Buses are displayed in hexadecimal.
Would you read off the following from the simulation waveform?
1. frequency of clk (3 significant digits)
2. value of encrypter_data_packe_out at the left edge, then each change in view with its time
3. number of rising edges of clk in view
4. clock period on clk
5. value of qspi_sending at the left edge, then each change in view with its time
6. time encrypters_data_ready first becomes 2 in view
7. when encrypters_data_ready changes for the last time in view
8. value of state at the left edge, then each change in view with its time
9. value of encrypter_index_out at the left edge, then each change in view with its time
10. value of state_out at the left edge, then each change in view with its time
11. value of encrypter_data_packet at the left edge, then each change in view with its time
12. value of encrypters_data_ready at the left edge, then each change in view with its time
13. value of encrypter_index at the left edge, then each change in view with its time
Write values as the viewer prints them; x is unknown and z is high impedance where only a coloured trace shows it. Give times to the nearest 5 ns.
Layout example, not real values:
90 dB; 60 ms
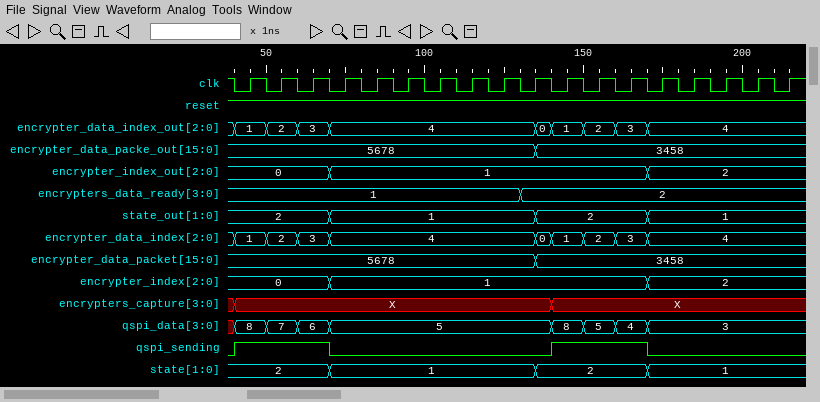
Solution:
100 MHz; 5678, 3458 at 135 ns; 18; 10 ns; 0, 1 at 40 ns, 0 at 70 ns, 1 at 140 ns, 0 at 170 ns; 130 ns; 130 ns; 2, 1 at 70 ns, 2 at 135 ns, 1 at 170 ns; 0, 1 at 70 ns, 2 at 170 ns; 2, 1 at 70 ns, 2 at 135 ns, 1 at 170 ns; 5678, 3458 at 135 ns; 1, 2 at 130 ns; 0, 1 at 70 ns, 2 at 170 ns
